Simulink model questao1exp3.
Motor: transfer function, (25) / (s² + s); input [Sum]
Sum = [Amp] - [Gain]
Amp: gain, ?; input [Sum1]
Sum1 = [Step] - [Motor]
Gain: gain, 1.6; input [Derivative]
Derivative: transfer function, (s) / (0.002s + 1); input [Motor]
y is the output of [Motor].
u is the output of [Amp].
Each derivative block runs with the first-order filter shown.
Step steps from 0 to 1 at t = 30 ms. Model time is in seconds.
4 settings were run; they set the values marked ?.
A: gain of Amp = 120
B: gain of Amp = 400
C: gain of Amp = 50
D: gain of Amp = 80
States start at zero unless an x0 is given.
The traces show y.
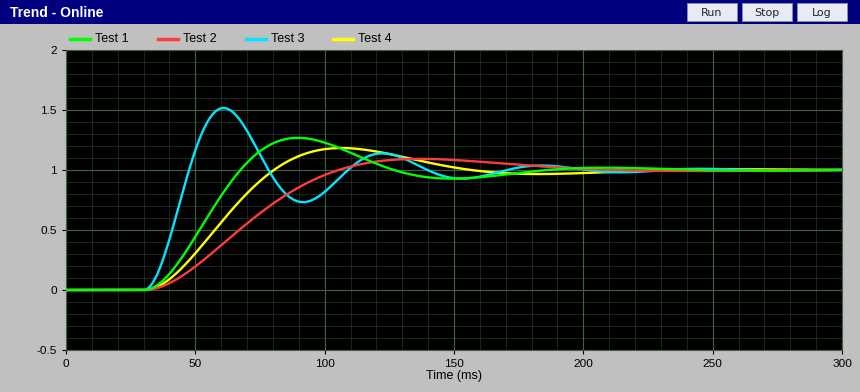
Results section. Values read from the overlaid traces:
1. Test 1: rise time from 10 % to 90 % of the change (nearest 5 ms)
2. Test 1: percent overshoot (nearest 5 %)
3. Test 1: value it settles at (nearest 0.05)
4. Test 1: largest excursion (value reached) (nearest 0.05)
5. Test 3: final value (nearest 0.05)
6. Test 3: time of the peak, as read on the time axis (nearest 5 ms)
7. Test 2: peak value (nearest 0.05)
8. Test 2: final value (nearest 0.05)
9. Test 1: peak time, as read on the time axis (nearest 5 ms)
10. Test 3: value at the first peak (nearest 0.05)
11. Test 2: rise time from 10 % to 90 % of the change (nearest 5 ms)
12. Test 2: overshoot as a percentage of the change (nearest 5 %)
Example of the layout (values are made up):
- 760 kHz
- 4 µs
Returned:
- 25 ms
- 25 %
- 1.00
- 1.25
- 1.00
- 60 ms
- 1.10
- 1.00
- 90 ms
- 1.50
- 50 ms
- 10 %
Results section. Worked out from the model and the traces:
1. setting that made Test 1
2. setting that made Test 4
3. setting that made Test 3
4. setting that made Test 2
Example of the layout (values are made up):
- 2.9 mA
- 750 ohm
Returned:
- A
- D
- B
- C
